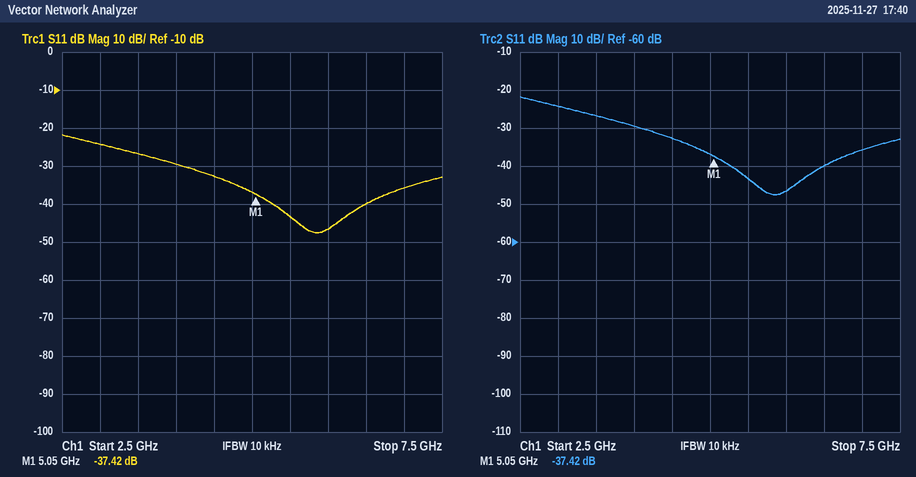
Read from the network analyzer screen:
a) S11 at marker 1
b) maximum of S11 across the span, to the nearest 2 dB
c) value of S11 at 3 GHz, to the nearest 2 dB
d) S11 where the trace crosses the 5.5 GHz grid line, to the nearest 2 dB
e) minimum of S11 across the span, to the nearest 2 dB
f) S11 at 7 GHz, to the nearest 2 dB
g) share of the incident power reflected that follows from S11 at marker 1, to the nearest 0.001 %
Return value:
-37.42 dB
-22 dB
-24 dB
-44 dB
-48 dB
-36 dB
0.018 %
